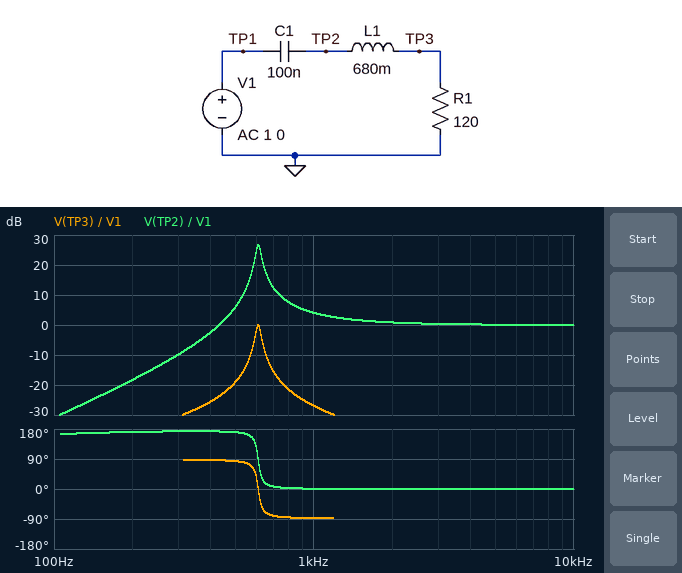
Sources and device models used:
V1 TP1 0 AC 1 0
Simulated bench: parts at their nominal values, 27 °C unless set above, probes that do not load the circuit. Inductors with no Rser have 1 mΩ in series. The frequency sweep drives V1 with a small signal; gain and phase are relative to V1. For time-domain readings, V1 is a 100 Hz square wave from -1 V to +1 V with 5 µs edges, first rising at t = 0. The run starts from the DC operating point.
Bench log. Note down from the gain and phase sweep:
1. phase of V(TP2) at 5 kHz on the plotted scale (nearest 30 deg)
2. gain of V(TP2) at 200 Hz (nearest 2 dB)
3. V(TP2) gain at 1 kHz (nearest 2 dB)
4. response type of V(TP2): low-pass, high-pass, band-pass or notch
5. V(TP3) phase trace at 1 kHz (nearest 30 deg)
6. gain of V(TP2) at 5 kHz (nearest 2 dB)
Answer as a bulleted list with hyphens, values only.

- 0 deg
- -18 dB
- 4 dB
- high-pass
- -90 deg
- 0 dB
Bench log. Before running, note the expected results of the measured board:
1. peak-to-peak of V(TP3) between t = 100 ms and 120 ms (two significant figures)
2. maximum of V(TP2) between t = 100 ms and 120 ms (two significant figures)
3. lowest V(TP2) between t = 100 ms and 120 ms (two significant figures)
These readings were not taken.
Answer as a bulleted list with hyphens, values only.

- 110 mV
- 1.2 V
- -1.2 V
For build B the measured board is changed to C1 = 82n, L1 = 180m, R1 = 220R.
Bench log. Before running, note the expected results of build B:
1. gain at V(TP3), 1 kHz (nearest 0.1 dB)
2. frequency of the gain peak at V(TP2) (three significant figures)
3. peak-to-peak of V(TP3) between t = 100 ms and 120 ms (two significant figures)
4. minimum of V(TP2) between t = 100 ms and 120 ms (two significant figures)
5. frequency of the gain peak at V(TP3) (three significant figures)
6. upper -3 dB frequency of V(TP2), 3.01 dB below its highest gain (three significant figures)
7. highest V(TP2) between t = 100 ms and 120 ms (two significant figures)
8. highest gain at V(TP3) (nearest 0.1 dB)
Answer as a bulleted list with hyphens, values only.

- -11.6 dB
- 1.32 kHz
- 560 mV
- -2.1 V
- 1.31 kHz
- 1.43 kHz
- 2.1 V
- 0 dB
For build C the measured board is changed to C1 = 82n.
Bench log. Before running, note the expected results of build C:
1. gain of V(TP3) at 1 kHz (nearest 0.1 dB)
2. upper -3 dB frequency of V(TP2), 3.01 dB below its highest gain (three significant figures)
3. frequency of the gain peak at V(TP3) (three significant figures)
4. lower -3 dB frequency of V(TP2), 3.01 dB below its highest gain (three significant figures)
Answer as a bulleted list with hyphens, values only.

- -25.8 dB
- 689 Hz
- 674 Hz
- 661 Hz
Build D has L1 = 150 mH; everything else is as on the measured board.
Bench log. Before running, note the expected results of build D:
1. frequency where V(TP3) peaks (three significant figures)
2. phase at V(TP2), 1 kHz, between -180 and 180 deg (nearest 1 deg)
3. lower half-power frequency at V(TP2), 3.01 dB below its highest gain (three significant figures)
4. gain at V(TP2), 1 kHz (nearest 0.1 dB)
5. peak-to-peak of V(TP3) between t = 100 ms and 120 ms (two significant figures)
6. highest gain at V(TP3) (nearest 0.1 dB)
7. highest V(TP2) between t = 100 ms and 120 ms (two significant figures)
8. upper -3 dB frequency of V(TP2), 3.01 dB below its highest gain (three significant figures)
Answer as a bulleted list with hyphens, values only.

- 1.30 kHz
- 162 deg
- 1.24 kHz
- 3.2 dB
- 420 mV
- 0 dB
- 2.3 V
- 1.37 kHz
